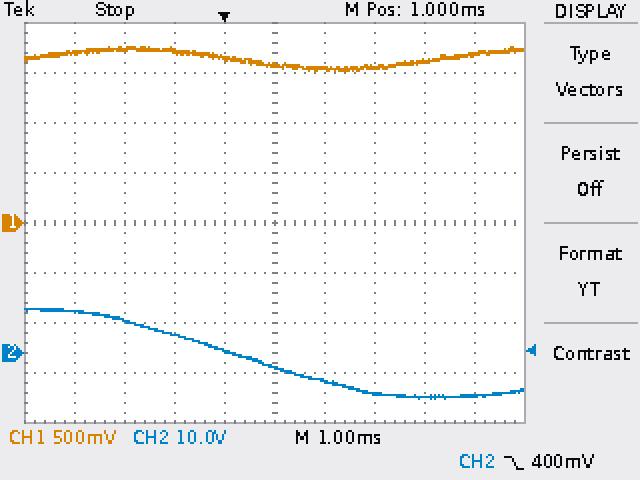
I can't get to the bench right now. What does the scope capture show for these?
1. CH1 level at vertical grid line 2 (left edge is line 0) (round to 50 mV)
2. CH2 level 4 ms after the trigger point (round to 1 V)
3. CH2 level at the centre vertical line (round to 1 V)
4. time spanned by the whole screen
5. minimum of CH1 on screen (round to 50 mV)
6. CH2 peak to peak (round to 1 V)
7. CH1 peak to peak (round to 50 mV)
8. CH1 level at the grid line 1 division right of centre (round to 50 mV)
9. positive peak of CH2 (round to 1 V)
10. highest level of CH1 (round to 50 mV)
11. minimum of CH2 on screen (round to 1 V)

1.75 V
-9 V
-3 V
10 ms
1.50 V
18 V
250 mV
1.55 V
9 V
1.75 V
-9 V
